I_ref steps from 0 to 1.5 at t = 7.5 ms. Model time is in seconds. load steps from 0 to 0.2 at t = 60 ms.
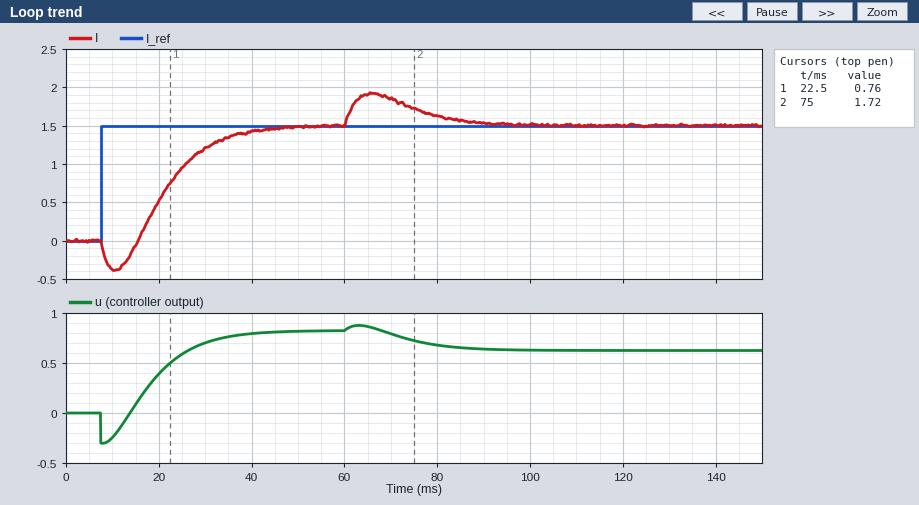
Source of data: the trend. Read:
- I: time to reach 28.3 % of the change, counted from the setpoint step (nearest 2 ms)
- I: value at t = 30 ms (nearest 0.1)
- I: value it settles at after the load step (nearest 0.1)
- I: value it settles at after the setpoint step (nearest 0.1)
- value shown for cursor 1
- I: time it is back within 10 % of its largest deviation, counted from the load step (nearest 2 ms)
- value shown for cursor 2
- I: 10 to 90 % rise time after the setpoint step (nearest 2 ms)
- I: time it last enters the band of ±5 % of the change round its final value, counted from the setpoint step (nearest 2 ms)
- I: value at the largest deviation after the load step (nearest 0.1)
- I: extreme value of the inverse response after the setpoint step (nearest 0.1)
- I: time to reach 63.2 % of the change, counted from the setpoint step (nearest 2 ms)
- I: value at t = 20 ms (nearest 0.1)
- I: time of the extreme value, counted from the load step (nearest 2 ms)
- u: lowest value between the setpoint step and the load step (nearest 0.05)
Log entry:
12 ms
1.2
1.5
1.5
0.76
28 ms
1.72
18 ms
32 ms
1.9
-0.4
18 ms
0.5
6 ms
-0.30
